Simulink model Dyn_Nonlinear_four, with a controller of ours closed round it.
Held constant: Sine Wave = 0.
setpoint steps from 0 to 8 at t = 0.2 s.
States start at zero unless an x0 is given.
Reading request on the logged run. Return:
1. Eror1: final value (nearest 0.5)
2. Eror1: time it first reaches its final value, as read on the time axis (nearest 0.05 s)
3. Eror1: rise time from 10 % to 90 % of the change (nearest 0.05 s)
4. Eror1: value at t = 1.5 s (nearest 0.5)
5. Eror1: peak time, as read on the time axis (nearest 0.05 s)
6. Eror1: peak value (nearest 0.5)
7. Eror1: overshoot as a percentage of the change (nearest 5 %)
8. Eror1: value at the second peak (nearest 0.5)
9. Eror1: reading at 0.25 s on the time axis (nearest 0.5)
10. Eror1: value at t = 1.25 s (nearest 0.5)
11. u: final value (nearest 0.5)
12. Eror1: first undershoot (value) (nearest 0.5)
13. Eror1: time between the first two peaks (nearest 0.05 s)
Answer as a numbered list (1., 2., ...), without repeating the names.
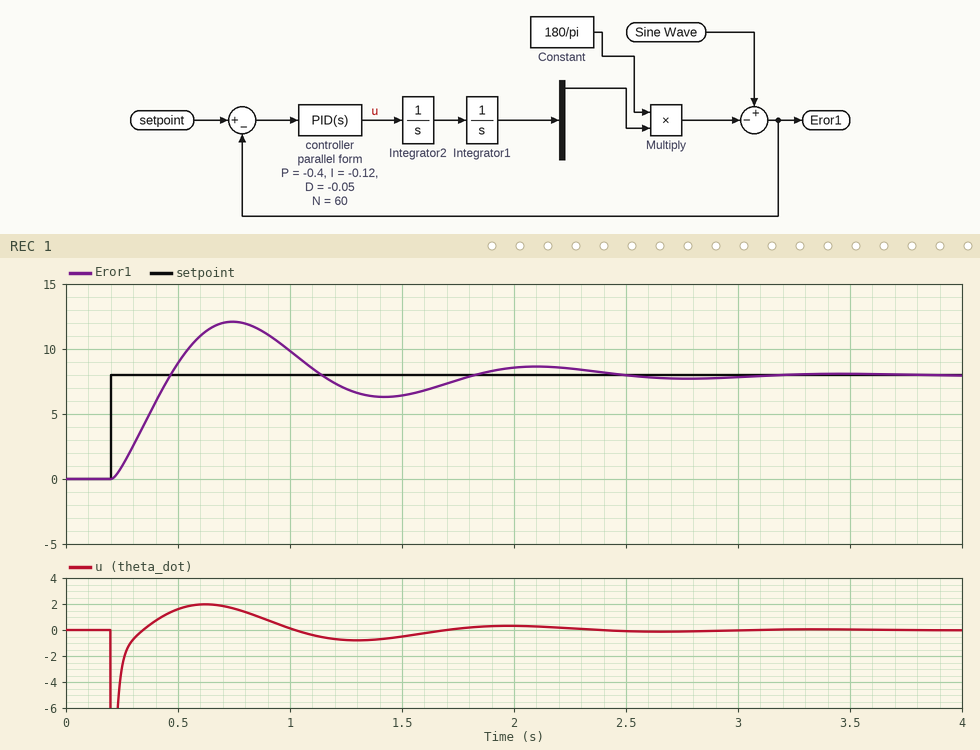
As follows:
1. 8.0
2. 0.45 s
3. 0.20 s
4. 6.5
5. 0.75 s
6. 12.0
7. 50 %
8. 8.5
9. 1.0
10. 7.0
11. 0.0
12. 6.5
13. 1.35 s
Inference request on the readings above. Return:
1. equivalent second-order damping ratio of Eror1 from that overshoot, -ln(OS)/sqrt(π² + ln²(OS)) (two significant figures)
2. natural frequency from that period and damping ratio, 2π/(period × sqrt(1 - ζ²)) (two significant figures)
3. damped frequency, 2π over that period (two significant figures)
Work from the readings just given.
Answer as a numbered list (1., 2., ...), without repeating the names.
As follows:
1. 0.22
2. 4.8 rad/s
3. 4.7 rad/s
